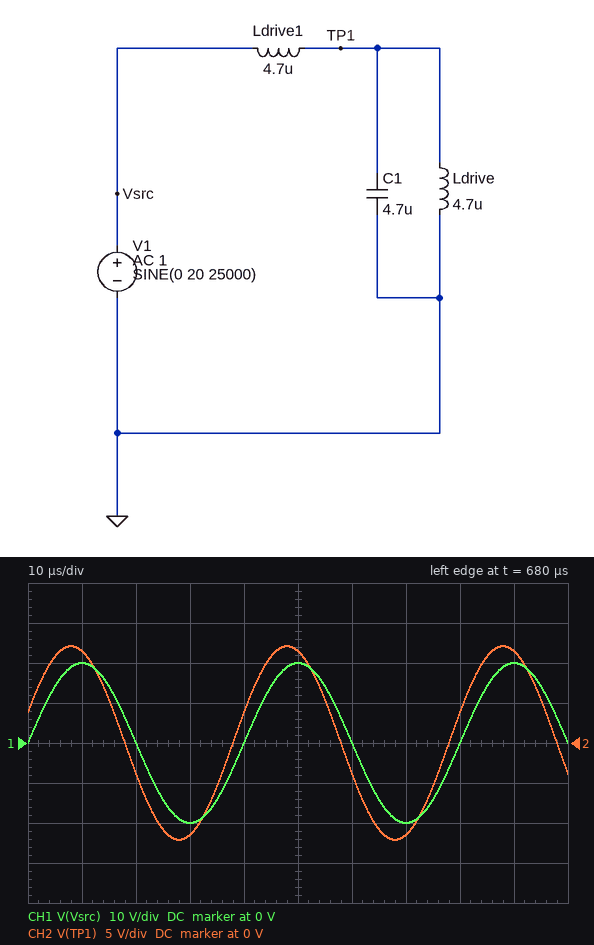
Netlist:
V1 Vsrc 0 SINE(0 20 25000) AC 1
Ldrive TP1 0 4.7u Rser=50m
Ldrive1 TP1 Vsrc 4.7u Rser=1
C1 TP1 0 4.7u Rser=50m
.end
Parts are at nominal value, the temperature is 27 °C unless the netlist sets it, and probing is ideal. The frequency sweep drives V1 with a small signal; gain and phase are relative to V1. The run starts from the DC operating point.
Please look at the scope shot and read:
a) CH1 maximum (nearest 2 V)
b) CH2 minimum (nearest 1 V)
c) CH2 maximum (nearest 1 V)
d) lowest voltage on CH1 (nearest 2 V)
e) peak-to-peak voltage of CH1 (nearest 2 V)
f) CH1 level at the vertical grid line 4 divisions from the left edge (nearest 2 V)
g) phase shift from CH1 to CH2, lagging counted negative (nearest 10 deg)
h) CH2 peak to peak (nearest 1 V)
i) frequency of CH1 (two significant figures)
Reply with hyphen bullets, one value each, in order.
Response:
- 20 V
- -12 V
- 12 V
- -20 V
- 40 V
- 0 V
- 20 deg
- 24 V
- 25 kHz
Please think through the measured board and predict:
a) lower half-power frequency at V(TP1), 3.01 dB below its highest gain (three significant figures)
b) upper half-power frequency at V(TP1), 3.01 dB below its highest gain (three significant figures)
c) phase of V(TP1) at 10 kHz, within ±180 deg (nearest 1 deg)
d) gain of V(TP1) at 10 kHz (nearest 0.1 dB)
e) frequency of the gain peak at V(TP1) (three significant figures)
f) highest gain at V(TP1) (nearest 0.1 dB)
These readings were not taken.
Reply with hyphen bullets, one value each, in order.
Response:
- 33.4 kHz
- 52.3 kHz
- 49 deg
- -11.5 dB
- 43.4 kHz
- 2.0 dB
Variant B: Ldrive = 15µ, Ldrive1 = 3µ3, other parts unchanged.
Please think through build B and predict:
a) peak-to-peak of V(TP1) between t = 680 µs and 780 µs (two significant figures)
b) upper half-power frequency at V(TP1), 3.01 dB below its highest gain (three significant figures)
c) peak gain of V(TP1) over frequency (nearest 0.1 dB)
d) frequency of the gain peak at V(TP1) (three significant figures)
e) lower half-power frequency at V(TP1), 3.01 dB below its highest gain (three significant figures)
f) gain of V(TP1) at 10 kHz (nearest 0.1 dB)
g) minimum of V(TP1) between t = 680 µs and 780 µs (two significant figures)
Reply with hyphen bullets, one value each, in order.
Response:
- 43 V
- 47.8 kHz
- 0.8 dB
- 30.2 kHz
- 12.0 kHz
- -3.1 dB
- -21 V
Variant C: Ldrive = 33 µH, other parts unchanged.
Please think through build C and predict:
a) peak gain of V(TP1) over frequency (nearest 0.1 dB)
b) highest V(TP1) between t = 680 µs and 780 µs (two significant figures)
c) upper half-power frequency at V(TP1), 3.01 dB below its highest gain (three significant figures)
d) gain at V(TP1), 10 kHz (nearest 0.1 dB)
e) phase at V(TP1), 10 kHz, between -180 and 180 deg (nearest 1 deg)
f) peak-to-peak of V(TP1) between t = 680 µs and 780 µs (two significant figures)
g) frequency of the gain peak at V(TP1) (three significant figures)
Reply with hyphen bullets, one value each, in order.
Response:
- 1.5 dB
- 24 V
- 40.7 kHz
- -0.7 dB
- 10 deg
- 47 V
- 26.7 kHz
